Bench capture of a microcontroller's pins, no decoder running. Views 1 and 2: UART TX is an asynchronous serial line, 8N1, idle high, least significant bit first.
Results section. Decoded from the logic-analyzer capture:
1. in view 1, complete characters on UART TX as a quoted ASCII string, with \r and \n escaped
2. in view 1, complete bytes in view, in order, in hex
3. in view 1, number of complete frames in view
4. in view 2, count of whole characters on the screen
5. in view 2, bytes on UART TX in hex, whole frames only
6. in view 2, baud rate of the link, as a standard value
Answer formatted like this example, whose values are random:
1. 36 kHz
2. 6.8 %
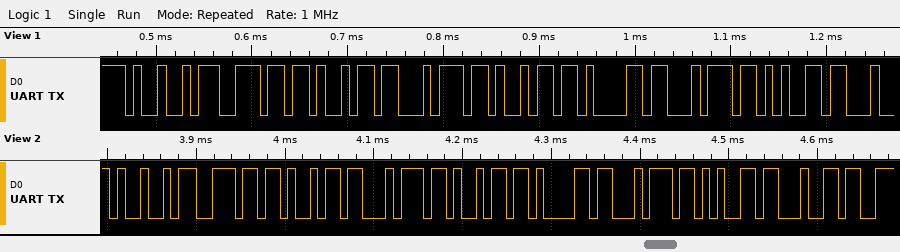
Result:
1. "Initiate"
2. 49 6E 69 74 69 61 74 65
3. 8
4. 9
5. 0x49 0x6E 0x69 0x74 0x69 0x61 0x74 0x65 0x64
6. 115200 baud
